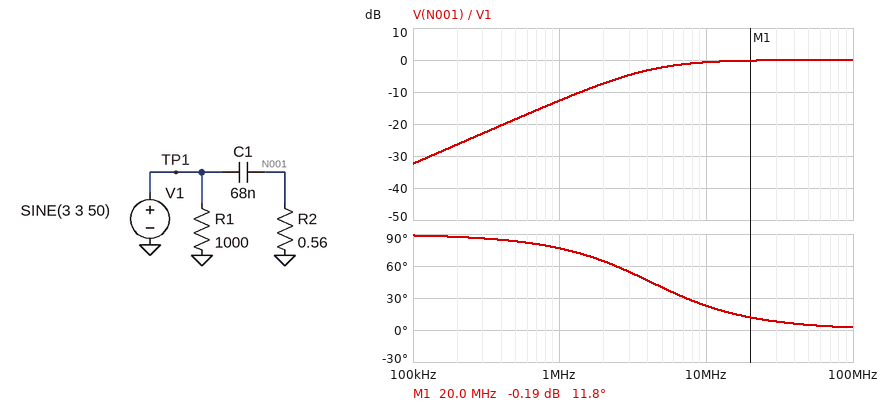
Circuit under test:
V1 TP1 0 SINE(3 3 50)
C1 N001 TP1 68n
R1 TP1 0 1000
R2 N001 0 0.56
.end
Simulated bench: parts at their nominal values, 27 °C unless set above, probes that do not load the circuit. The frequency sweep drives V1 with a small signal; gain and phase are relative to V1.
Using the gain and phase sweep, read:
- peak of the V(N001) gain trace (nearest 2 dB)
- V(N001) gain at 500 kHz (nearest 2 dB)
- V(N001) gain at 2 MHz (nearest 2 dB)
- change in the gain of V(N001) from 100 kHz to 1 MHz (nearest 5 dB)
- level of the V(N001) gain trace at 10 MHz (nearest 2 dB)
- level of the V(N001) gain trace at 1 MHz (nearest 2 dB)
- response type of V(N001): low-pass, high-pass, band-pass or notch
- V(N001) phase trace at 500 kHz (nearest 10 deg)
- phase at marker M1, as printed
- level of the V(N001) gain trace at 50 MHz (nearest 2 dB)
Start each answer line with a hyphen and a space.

- 0 dB
- -18 dB
- -8 dB
- 20 dB
- 0 dB
- -12 dB
- high-pass
- 80 deg
- 11.8 deg
- 0 dB
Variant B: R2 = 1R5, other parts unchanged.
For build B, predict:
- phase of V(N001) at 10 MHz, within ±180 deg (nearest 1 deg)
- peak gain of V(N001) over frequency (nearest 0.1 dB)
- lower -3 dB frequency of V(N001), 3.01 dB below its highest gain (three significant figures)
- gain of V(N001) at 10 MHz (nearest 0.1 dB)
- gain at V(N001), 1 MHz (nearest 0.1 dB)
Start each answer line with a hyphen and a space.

- 9 deg
- 0 dB
- 1.56 MHz
- -0.1 dB
- -5.4 dB
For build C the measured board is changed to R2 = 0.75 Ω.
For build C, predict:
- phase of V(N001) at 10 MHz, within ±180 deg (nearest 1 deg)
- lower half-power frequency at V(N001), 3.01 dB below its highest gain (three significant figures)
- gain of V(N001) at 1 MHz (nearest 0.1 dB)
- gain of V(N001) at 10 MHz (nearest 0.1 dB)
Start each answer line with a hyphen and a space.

- 17 deg
- 3.12 MHz
- -10.3 dB
- -0.4 dB
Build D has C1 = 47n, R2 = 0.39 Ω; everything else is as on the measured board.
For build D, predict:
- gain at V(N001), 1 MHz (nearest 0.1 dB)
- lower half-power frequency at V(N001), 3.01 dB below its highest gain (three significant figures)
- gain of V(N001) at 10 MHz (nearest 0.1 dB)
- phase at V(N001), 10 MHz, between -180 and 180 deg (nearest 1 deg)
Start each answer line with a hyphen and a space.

- -18.8 dB
- 8.68 MHz
- -2.4 dB
- 41 deg
